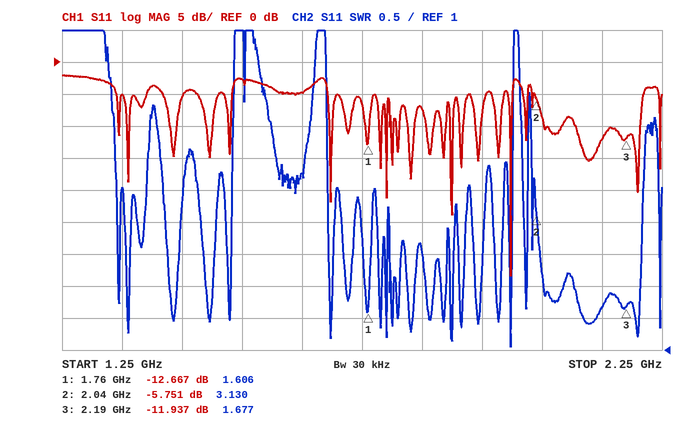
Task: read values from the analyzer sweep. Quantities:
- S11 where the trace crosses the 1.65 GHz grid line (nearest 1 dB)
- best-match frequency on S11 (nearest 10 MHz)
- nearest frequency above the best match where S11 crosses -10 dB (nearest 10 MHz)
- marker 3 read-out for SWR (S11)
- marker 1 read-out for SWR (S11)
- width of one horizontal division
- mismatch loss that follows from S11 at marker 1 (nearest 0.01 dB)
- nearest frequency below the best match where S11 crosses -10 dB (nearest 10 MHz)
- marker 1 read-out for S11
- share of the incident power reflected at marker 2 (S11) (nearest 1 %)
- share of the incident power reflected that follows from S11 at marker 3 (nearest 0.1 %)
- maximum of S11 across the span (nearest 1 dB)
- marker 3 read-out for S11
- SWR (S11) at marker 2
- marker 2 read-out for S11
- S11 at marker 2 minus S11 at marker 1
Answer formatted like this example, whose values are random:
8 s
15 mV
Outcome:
-5 dB
2.00 GHz
2.00 GHz
1.677
1.606
100 MHz
0.24 dB
2.00 GHz
-12.667 dB
27 %
6.4 %
-2 dB
-11.937 dB
3.130
-5.751 dB
6.916 dB
